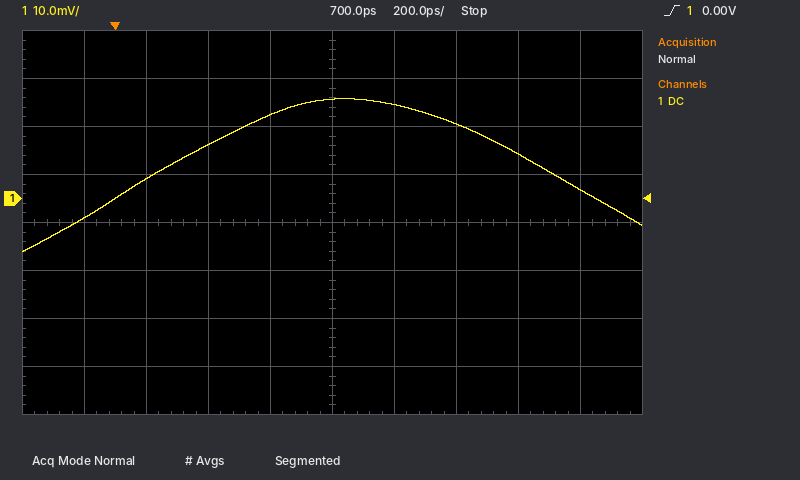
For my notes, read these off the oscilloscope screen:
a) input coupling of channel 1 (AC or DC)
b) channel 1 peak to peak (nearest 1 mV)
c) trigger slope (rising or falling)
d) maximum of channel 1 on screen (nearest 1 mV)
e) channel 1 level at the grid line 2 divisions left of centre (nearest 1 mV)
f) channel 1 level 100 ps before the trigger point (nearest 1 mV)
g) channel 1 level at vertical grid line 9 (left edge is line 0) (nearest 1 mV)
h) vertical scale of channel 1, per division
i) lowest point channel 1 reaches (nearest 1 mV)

DC
32 mV
rising
21 mV
11 mV
-4 mV
2 mV
10 mV
-11 mV
